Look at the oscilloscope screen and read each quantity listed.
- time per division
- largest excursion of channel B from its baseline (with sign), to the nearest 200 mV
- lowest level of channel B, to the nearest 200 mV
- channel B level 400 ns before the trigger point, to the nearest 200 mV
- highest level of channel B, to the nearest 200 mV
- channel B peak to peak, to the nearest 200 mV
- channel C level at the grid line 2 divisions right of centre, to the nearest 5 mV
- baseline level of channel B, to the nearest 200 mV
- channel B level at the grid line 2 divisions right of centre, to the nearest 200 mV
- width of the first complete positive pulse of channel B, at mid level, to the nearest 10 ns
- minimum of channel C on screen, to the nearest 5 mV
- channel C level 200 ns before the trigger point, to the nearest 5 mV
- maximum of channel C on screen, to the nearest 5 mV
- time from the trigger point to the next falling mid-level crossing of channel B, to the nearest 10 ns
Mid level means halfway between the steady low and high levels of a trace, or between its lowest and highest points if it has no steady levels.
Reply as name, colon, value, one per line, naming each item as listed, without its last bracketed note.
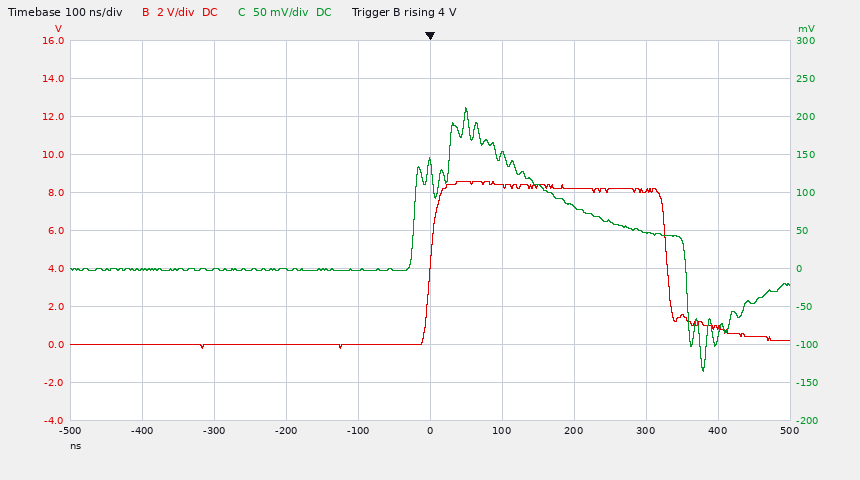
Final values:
time per division: 100 ns
largest excursion of channel B from its baseline (with sign), to the nearest 200 mV: +8.6 V
lowest level of channel B, to the nearest 200 mV: -200 mV
channel B level 400 ns before the trigger point, to the nearest 200 mV: 0.0 V
highest level of channel B, to the nearest 200 mV: 8.6 V
channel B peak to peak, to the nearest 200 mV: 8.8 V
channel C level at the grid line 2 divisions right of centre, to the nearest 5 mV: 80 mV
baseline level of channel B, to the nearest 200 mV: 0.0 V
channel B level at the grid line 2 divisions right of centre, to the nearest 200 mV: 8.2 V
width of the first complete positive pulse of channel B, at mid level, to the nearest 10 ns: 330 ns
minimum of channel C on screen, to the nearest 5 mV: -135 mV
channel C level 200 ns before the trigger point, to the nearest 5 mV: 0 mV
maximum of channel C on screen, to the nearest 5 mV: 210 mV
time from the trigger point to the next falling mid-level crossing of channel B, to the nearest 10 ns: 330 ns
